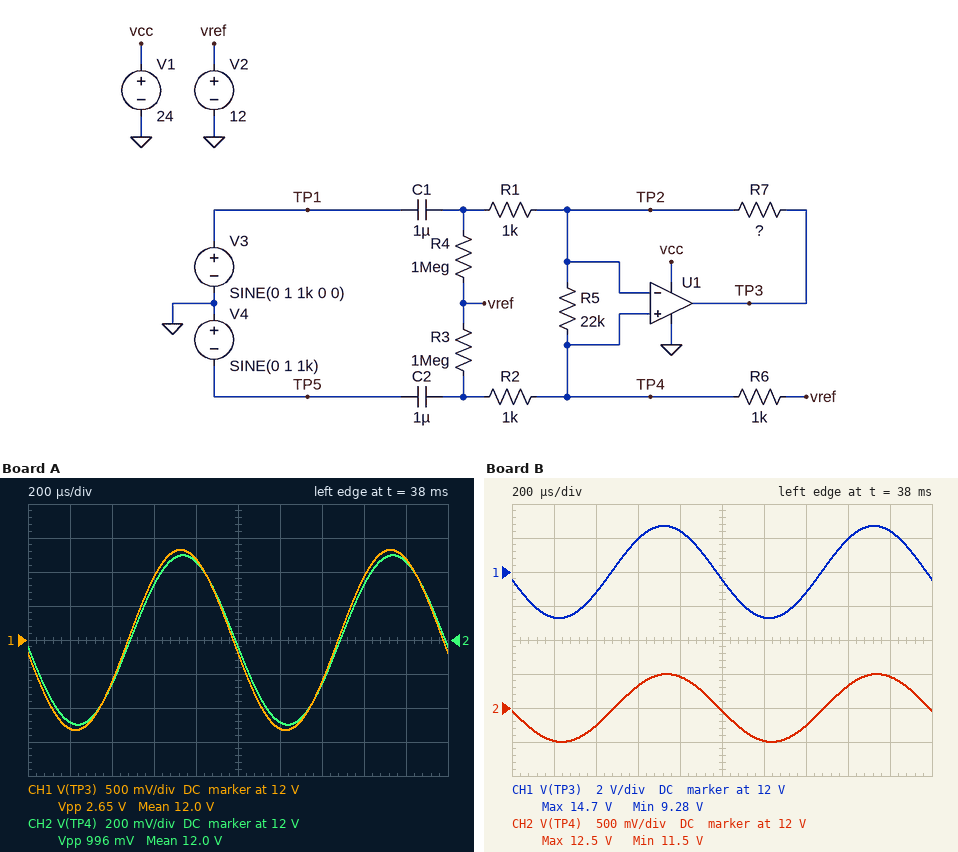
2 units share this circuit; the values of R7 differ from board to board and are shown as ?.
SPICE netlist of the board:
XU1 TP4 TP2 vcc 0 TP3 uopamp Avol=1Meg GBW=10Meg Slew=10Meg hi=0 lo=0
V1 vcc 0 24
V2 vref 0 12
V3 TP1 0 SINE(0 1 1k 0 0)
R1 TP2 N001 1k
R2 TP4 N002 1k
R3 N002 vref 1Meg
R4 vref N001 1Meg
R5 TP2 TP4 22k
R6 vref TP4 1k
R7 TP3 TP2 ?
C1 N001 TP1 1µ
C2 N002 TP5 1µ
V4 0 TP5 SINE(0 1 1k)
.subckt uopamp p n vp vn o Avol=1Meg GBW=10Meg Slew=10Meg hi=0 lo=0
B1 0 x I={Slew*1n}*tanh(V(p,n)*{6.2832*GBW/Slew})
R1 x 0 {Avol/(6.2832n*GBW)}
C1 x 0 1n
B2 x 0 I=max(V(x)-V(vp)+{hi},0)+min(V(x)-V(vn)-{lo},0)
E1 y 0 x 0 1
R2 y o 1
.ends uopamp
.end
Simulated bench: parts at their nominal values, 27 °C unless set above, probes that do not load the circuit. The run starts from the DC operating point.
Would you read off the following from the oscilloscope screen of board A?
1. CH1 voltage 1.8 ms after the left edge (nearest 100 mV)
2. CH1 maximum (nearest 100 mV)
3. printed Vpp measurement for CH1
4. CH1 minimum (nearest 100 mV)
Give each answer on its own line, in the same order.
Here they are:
13.2 V
13.3 V
2.65 V
10.7 V
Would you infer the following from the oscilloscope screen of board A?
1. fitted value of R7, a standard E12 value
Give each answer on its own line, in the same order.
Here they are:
560 Ω
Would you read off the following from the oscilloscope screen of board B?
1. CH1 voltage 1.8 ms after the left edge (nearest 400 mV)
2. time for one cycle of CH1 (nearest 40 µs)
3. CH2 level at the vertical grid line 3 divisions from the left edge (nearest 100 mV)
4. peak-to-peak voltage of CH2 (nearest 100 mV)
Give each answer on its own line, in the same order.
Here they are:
14.4 V
1.00 ms
12.3 V
1.0 V
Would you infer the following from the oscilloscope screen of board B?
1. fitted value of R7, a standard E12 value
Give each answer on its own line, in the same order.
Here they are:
1.5 kΩ
